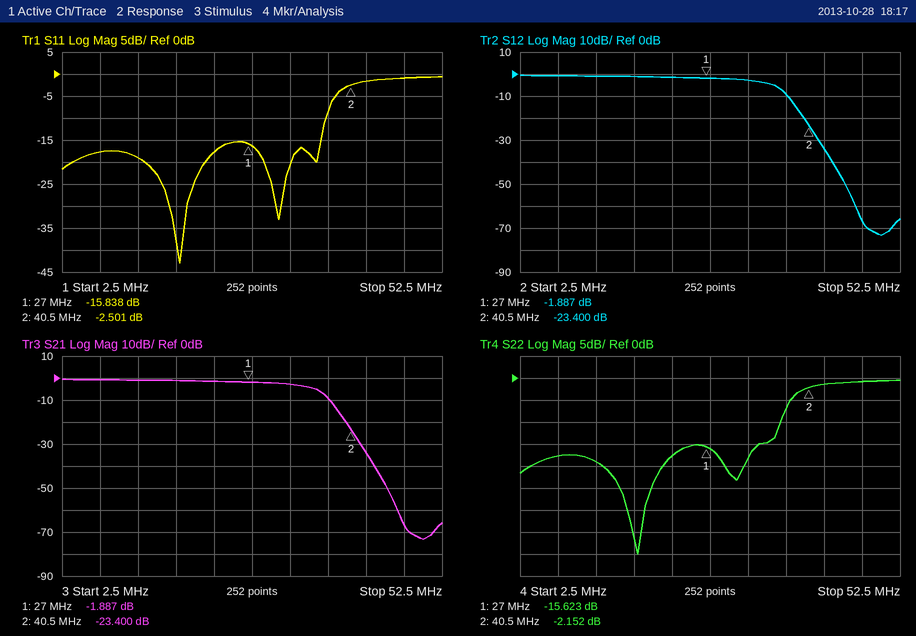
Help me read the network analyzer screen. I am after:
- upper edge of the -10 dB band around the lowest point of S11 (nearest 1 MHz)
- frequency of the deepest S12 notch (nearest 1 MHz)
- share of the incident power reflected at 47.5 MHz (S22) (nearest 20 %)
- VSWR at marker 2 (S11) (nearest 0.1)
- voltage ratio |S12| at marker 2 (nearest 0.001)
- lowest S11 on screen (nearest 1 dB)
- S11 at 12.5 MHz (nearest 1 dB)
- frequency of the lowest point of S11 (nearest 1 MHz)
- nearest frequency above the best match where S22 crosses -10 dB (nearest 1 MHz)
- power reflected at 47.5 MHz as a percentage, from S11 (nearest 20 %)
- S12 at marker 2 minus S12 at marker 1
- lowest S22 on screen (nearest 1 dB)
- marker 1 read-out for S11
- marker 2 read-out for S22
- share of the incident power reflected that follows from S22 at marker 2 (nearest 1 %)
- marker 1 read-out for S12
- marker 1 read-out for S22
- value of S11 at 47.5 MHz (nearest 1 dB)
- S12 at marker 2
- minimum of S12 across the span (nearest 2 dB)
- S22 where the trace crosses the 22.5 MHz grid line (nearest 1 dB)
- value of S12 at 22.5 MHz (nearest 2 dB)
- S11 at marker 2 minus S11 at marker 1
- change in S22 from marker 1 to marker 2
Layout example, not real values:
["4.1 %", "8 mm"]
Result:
["37 MHz", "50 MHz", "80 %", "7.0", "0.068", "-43 dB", "-19 dB", "18 MHz", "37 MHz", "80 %", "-21.513 dB", "-40 dB", "-15.838 dB", "-2.152 dB", "61 %", "-1.887 dB", "-15.623 dB", "-1 dB", "-23.400 dB", "-74 dB", "-18 dB", "-2 dB", "13.337 dB", "13.471 dB"]
